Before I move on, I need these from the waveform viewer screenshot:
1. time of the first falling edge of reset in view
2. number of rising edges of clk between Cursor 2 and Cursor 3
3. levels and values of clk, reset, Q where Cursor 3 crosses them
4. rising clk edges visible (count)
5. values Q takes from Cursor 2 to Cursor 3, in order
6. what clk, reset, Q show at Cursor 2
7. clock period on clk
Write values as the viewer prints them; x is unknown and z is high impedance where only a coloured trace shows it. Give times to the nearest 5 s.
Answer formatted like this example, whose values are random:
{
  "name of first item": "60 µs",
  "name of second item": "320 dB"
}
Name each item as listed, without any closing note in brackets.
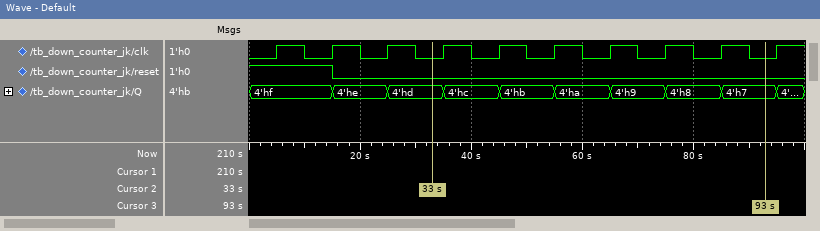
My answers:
{
  "time of the first falling edge of reset in view": "15 s",
  "number of rising edges of clk between Cursor 2 and Cursor 3": "6",
  "levels and values of clk, reset, Q where Cursor 3 crosses them": "clk=0, reset=0, Q=4'h7",
  "rising clk edges visible": "10",
  "values Q takes from Cursor 2 to Cursor 3, in order": "4'hd, 4'hc, 4'hb, 4'ha, 4'h9, 4'h8, 4'h7",
  "what clk, reset, Q show at Cursor 2": "clk=0, reset=0, Q=4'hd",
  "clock period on clk": "10 s"
}
